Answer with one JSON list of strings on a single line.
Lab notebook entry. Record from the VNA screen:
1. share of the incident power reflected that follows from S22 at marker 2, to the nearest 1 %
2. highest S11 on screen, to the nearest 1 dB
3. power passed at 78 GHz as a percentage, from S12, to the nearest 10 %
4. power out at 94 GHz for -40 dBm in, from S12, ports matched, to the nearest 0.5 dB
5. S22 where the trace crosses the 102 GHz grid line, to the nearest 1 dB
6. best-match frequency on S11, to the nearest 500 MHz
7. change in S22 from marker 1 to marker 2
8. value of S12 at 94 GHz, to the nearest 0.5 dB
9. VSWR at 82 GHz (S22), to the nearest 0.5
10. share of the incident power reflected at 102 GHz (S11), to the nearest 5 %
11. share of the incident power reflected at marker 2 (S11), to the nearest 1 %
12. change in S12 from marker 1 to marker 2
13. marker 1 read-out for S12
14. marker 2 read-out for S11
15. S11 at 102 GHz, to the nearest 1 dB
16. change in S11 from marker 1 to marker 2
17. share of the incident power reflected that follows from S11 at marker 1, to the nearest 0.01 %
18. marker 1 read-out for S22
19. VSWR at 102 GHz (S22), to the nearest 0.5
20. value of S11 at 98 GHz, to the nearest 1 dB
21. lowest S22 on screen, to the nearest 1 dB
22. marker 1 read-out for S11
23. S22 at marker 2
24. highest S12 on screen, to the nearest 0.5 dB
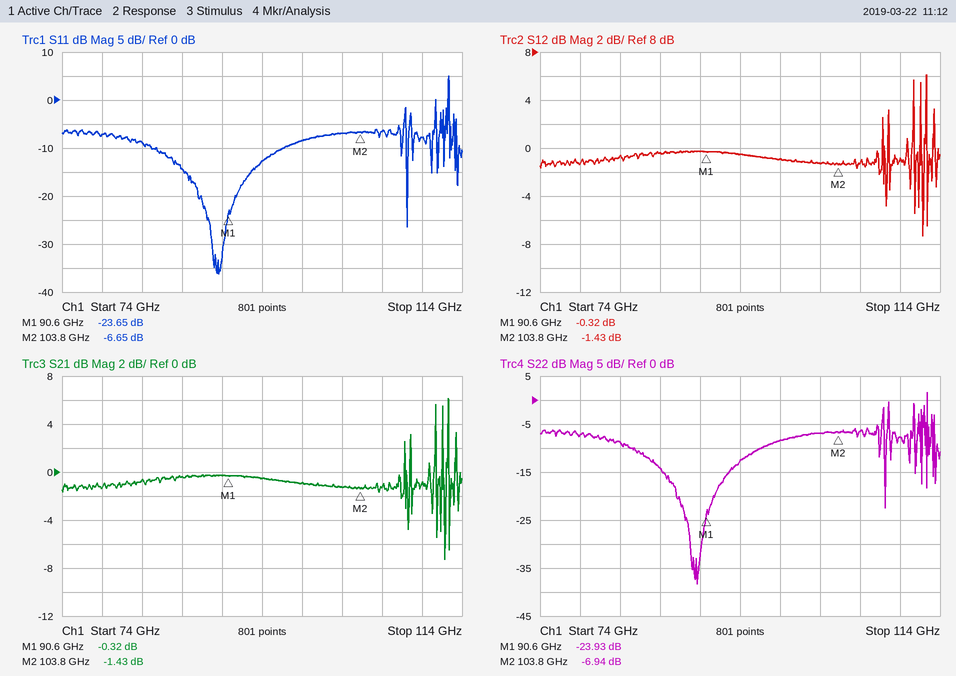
["20 %", "5 dB", "70 %", "-40.5 dBm", "-7 dB", "89.5 GHz", "16.99 dB", "-0.5 dB", "2.0", "20 %", "22 %", "-1.11 dB", "-0.32 dB", "-6.65 dB", "-7 dB", "17.00 dB", "0.43 %", "-23.93 dB", "2.5", "-8 dB", "-38 dB", "-23.65 dB", "-6.94 dB", "6.0 dB"]
